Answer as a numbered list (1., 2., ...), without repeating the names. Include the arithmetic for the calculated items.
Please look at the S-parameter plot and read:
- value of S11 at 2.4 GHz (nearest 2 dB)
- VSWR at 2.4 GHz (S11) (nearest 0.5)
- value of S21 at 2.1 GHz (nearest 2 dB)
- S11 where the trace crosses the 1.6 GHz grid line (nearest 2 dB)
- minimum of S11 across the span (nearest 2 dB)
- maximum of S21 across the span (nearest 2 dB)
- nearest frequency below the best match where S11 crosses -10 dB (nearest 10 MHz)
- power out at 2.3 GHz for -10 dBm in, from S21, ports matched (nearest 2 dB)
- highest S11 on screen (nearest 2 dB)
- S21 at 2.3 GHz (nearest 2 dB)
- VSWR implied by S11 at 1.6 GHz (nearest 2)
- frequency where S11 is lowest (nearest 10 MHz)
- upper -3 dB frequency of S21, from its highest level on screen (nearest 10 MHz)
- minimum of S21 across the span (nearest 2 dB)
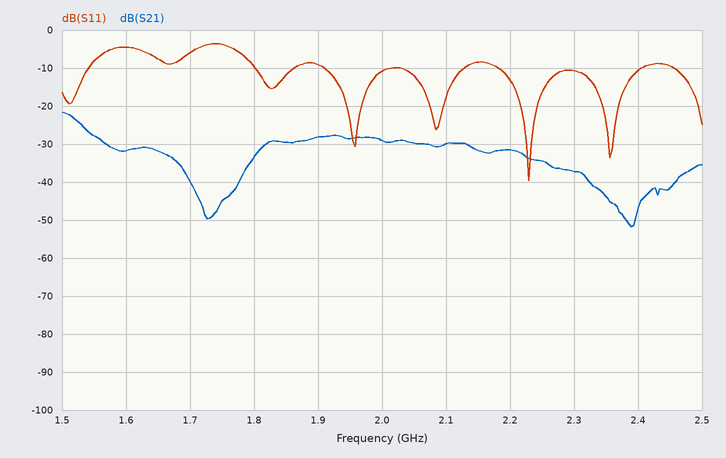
1. -10 dB
2. |Γ| = 10^(-10/20) = 0.3162; VSWR = (1 + 0.3162)/(1 − 0.3162) ≈ 1.92, so 2.0 to the nearest 0.5
3. -30 dB
4. -4 dB
5. -40 dB
6. -22 dB
7. 2.18 GHz
8. -10 dBm + (-38 dB) = -48 dBm
9. -4 dB
10. -38 dB
11. |Γ| = 10^(-4/20) = 0.6310; VSWR = (1 + 0.6310)/(1 − 0.6310) ≈ 4
12. 2.23 GHz
13. 1.53 GHz
14. -52 dB
